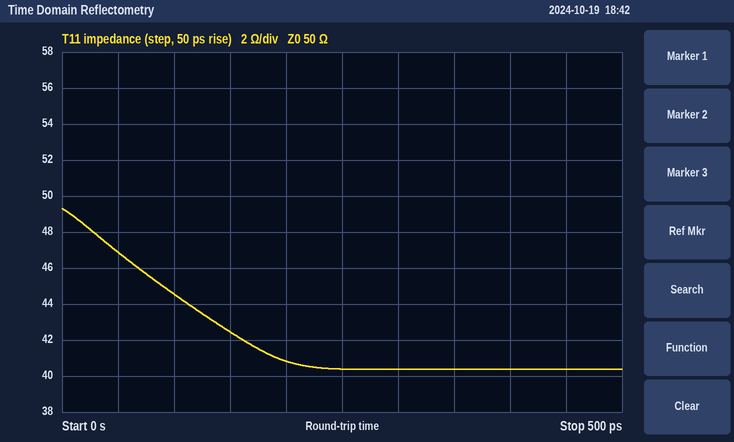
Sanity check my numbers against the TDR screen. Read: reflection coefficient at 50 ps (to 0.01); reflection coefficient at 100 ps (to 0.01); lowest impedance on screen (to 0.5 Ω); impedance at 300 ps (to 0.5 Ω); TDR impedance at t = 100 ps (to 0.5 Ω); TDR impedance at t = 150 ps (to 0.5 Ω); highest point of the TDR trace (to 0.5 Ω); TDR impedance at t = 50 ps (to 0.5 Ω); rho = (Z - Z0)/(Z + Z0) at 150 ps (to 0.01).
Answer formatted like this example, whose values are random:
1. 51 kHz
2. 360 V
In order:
1. -0.03
2. -0.06
3. 40.5 Ω
4. 40.5 Ω
5. 44.5 Ω
6. 42.5 Ω
7. 49.5 Ω
8. 47.0 Ω
9. -0.08
